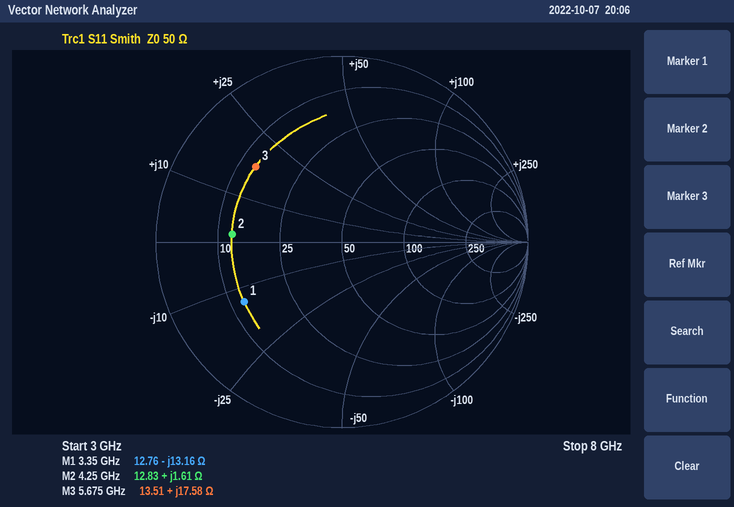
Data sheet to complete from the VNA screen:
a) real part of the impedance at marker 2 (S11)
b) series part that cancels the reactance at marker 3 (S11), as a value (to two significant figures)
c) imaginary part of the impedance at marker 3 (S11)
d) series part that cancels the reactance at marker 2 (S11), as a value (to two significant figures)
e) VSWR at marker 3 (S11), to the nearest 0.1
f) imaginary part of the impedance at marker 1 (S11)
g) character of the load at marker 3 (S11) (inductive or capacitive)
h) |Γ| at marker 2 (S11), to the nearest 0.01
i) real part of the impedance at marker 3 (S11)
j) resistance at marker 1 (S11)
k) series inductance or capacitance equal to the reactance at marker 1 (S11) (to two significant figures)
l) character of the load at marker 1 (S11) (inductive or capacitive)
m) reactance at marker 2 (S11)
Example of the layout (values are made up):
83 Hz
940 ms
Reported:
12.83 Ω
1.6 pF
+17.58 Ω
23 pF
4.2
-13.16 Ω
inductive
0.59
13.51 Ω
12.76 Ω
3.6 pF
capacitive
+1.61 Ω
